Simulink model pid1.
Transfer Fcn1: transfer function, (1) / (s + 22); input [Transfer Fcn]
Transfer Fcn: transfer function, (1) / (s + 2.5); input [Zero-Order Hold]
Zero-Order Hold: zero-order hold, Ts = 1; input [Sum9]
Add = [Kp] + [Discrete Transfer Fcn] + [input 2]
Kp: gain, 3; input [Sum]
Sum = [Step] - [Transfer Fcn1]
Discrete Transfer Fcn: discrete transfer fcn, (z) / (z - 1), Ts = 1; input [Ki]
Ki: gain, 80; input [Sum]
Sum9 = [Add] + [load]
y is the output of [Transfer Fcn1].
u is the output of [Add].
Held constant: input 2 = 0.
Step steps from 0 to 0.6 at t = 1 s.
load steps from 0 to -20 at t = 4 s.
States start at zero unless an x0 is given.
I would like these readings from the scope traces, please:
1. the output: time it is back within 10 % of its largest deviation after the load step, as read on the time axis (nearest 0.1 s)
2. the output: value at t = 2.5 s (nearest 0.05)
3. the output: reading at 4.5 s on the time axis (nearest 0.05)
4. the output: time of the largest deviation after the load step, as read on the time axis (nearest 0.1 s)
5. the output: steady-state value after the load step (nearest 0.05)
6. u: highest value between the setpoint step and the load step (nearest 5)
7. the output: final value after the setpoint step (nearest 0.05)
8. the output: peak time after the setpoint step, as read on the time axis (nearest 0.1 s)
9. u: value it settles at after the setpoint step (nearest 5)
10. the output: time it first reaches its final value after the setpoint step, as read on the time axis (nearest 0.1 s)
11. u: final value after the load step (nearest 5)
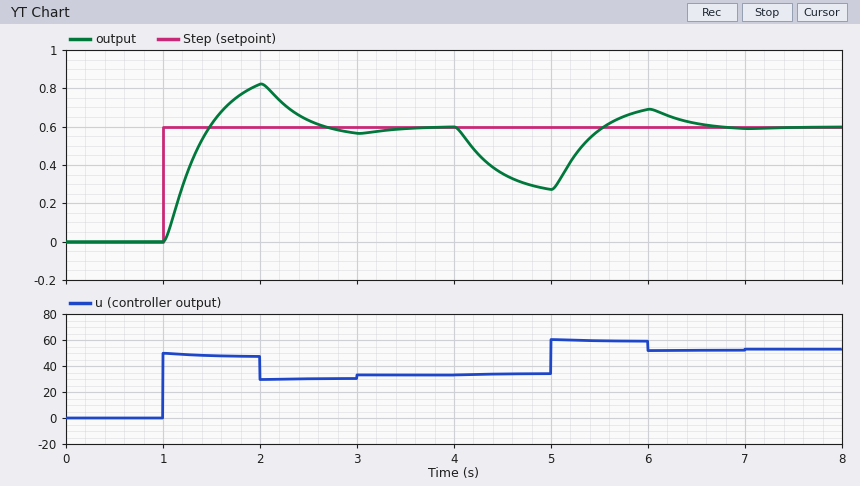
6.4 s
0.65
0.35
5.0 s
0.60
50
0.60
2.0 s
35
1.5 s
55
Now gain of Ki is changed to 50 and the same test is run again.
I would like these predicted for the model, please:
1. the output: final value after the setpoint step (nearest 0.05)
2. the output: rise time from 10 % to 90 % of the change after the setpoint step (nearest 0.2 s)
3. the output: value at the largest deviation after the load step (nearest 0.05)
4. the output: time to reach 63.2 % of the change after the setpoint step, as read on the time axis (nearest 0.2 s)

0.60
1.0 s
0.25
1.4 s
